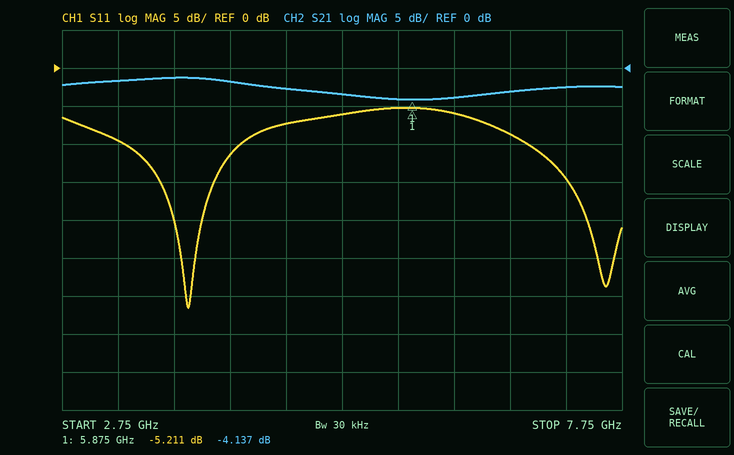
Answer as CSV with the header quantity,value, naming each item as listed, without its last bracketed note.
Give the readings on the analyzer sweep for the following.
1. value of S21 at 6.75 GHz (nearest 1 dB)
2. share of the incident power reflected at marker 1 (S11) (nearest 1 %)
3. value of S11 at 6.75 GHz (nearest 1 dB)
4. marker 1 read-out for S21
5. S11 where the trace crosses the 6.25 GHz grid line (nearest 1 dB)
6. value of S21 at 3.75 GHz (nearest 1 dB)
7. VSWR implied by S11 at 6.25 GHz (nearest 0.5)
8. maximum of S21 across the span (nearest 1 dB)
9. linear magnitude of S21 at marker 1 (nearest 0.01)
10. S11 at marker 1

quantity,value
value of S21 at 6.75 GHz,-3 dB
share of the incident power reflected at marker 1 (S11),30 %
value of S11 at 6.75 GHz,-9 dB
marker 1 read-out for S21,-4.137 dB
S11 where the trace crosses the 6.25 GHz grid line,-6 dB
value of S21 at 3.75 GHz,-1 dB
VSWR implied by S11 at 6.25 GHz,3.0
maximum of S21 across the span,-1 dB
linear magnitude of S21 at marker 1,0.62
S11 at marker 1,-5.211 dB
